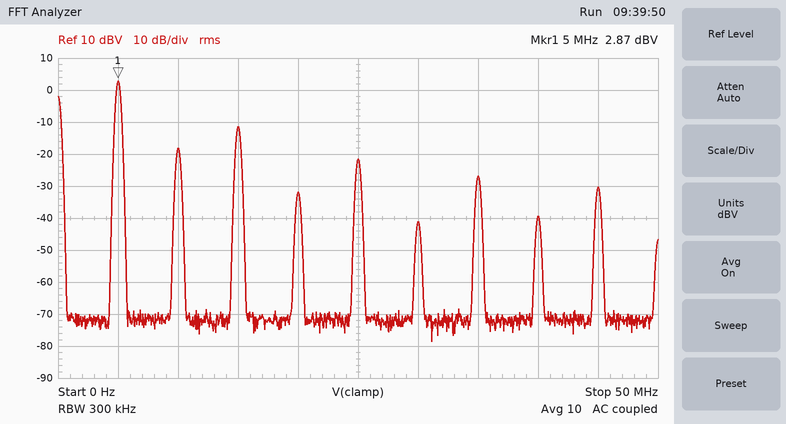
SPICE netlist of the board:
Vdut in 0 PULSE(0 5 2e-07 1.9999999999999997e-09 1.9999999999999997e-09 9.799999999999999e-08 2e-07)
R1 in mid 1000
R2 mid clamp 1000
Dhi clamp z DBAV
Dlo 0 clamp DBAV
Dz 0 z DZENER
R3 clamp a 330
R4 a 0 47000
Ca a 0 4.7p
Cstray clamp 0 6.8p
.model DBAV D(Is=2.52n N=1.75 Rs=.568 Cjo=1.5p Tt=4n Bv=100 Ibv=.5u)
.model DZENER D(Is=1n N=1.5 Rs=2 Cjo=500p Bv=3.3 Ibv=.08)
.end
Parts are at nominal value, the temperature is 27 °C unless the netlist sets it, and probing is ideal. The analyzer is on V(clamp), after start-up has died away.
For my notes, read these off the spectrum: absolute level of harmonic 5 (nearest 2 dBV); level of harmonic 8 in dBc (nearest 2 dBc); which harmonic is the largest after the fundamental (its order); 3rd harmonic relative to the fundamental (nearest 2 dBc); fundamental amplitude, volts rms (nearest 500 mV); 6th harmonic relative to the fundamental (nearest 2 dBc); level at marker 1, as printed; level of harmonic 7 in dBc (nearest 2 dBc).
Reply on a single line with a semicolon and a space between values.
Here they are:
-22 dBV; -42 dBc; 3; -14 dBc; 1.5 V; -44 dBc; 2.87 dBV; -30 dBc
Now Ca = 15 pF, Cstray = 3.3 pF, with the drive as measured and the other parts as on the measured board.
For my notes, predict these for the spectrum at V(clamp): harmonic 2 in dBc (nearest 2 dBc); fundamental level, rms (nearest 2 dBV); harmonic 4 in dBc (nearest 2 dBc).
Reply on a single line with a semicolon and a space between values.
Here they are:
-22 dBc; 2 dBV; -40 dBc
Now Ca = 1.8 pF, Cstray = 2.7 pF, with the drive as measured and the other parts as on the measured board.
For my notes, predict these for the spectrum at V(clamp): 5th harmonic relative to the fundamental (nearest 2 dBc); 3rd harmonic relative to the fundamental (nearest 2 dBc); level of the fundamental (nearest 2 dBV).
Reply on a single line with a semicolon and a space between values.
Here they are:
-18 dBc; -12 dBc; 4 dBV
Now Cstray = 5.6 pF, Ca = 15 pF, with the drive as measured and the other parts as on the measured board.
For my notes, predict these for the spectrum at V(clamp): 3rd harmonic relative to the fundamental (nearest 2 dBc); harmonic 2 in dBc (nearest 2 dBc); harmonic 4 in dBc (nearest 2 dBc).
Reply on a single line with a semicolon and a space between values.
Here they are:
-18 dBc; -24 dBc; -38 dBc
